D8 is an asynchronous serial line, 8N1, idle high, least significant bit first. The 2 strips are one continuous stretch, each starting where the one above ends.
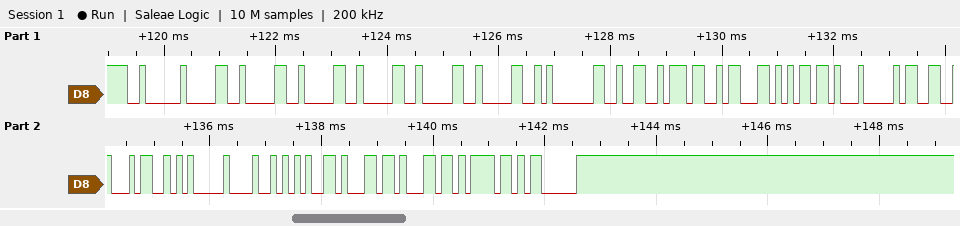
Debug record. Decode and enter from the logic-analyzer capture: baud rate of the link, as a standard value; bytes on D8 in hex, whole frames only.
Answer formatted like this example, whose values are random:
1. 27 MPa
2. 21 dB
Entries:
1. 9600 baud
2. 02 30 30 30 30 30 30 01 32 37 63 6D 04 33 34 05 48 65 6C 6C 6F 03
